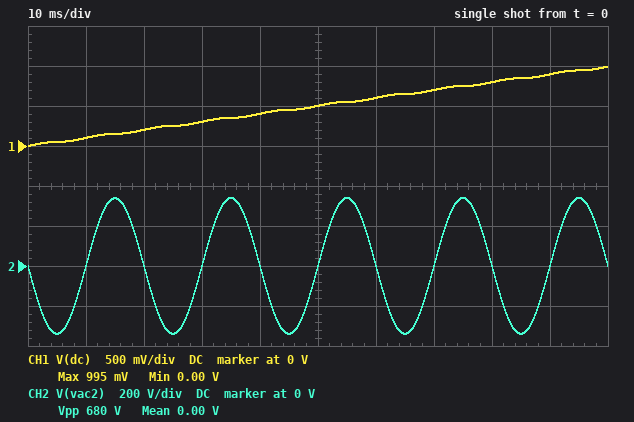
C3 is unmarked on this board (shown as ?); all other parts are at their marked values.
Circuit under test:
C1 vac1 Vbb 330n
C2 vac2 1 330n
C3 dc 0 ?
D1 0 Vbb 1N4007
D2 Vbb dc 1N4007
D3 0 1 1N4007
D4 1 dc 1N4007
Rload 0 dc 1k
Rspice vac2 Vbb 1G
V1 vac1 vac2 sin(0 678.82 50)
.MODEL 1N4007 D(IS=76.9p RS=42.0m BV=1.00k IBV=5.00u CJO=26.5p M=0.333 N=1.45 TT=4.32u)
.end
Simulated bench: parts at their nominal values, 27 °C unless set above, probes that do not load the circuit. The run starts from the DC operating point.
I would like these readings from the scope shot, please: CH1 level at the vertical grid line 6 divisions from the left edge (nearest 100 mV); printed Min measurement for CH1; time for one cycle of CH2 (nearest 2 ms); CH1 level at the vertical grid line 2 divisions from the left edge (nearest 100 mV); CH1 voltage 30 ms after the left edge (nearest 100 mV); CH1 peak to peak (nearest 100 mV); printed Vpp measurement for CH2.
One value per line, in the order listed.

600 mV
0.00 V
20 ms
200 mV
300 mV
1.0 V
680 V
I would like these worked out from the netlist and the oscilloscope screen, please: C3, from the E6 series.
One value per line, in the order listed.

2.2 mF
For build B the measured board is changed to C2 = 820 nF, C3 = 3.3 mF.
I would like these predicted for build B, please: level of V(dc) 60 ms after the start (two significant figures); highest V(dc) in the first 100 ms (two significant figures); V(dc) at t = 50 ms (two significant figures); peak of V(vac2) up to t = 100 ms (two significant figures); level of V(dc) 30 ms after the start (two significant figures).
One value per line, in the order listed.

570 mV
950 mV
480 mV
200 V
290 mV
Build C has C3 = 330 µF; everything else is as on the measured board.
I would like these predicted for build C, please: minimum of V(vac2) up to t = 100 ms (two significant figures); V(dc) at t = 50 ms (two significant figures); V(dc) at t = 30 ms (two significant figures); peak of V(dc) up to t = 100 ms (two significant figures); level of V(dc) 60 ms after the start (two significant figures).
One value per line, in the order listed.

-340 V
3.1 V
1.9 V
5.8 V
3.7 V
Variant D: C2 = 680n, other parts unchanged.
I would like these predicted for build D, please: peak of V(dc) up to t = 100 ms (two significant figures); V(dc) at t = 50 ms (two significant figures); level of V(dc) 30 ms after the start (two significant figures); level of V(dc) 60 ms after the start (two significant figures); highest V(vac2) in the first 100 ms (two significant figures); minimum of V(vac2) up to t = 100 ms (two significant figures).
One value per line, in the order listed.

1.3 V
680 mV
410 mV
810 mV
220 V
-220 V
